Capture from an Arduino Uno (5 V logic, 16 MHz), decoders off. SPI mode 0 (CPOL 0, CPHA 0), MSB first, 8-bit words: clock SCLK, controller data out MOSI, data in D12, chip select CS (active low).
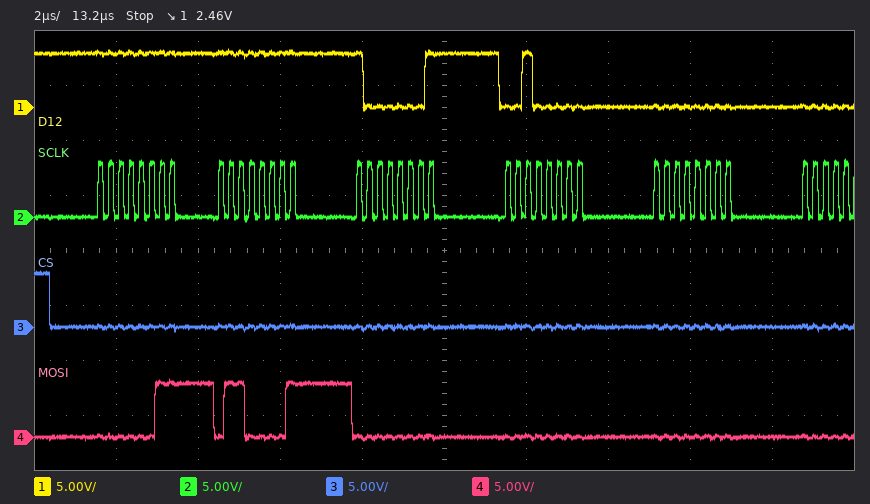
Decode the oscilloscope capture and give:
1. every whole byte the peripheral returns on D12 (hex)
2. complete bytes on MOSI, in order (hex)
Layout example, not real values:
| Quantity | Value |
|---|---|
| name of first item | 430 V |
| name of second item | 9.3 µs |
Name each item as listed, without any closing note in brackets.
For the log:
| Quantity | Value |
|---|---|
| every whole byte the peripheral returns on D12 | FF FF 81 20 00 |
| complete bytes on MOSI, in order | 03 61 00 00 00 |
